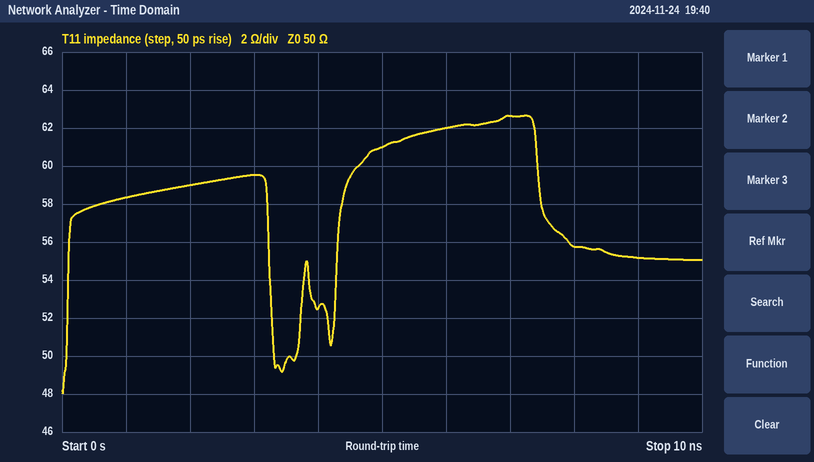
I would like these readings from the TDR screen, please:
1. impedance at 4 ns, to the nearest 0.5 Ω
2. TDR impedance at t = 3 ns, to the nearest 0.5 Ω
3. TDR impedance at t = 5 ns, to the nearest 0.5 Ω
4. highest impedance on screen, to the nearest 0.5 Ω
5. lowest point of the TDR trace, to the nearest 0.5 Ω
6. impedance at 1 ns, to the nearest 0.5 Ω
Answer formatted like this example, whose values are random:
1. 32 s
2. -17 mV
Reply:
1. 52.5 Ω
2. 59.5 Ω
3. 61.0 Ω
4. 62.5 Ω
5. 48.0 Ω
6. 58.5 Ω
